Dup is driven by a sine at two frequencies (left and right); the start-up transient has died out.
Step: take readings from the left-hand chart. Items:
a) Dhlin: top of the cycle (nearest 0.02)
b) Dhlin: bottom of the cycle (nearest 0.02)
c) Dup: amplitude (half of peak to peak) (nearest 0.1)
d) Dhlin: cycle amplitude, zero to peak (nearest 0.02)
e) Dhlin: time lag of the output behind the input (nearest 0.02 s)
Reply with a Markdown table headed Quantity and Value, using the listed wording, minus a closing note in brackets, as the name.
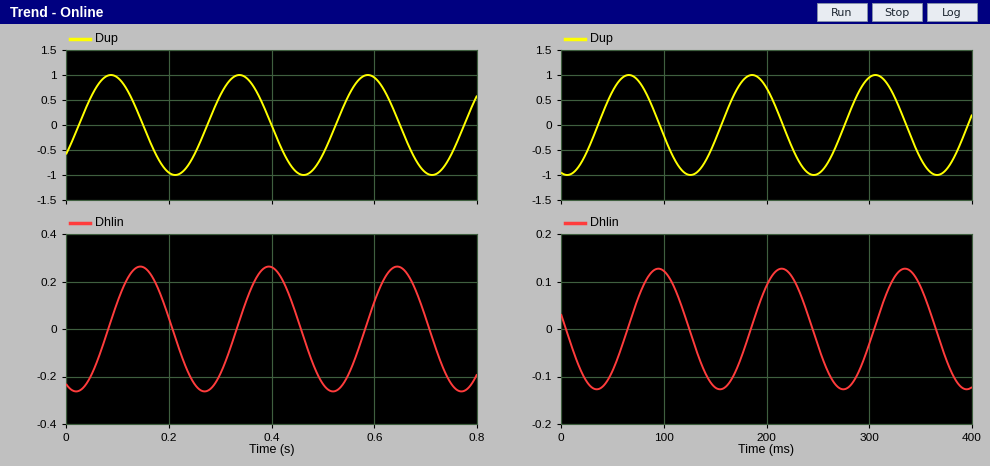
| Quantity | Value |
|---|---|
| Dhlin: top of the cycle | 0.26 |
| Dhlin: bottom of the cycle | -0.26 |
| Dup: amplitude (half of peak to peak) | 1.0 |
| Dhlin: cycle amplitude, zero to peak | 0.26 |
| Dhlin: time lag of the output behind the input | 0.06 s |
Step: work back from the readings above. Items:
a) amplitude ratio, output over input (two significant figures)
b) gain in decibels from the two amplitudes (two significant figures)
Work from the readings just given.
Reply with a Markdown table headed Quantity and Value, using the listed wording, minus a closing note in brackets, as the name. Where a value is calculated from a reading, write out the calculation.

| Quantity | Value |
|---|---|
| amplitude ratio, output over input | 0.26 / 1 = 0.26 |
| gain in decibels from the two amplitudes | 20 log10(0.26 / 1) = -12 dB |
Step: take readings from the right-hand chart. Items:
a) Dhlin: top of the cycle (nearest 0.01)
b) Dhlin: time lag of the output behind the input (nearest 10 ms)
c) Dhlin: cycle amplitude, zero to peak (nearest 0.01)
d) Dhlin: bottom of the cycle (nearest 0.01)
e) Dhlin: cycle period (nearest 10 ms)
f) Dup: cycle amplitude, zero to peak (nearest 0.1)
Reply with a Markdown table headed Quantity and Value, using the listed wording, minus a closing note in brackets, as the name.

| Quantity | Value |
|---|---|
| Dhlin: top of the cycle | 0.13 |
| Dhlin: time lag of the output behind the input | 30 ms |
| Dhlin: cycle amplitude, zero to peak | 0.13 |
| Dhlin: bottom of the cycle | -0.13 |
| Dhlin: cycle period | 120 ms |
| Dup: cycle amplitude, zero to peak | 1.0 |
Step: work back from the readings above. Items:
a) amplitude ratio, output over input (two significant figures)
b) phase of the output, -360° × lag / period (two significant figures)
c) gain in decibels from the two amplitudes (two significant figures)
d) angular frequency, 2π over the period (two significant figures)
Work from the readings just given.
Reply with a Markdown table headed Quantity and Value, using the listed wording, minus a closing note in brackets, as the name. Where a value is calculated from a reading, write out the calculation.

| Quantity | Value |
|---|---|
| amplitude ratio, output over input | 0.13 / 1 = 0.13 |
| phase of the output, -360° × lag / period | -360 × 30 / 120 = -90° |
| gain in decibels from the two amplitudes | 20 log10(0.13 / 1) = -18 dB |
| angular frequency, 2π over the period | 2π / 120 = 0.052 rad/ms |
